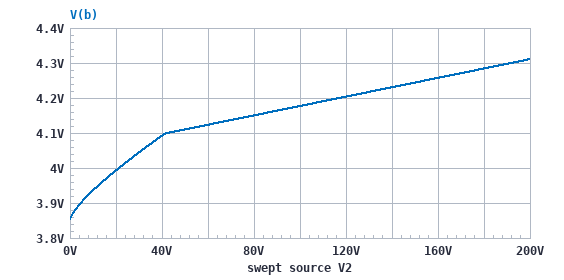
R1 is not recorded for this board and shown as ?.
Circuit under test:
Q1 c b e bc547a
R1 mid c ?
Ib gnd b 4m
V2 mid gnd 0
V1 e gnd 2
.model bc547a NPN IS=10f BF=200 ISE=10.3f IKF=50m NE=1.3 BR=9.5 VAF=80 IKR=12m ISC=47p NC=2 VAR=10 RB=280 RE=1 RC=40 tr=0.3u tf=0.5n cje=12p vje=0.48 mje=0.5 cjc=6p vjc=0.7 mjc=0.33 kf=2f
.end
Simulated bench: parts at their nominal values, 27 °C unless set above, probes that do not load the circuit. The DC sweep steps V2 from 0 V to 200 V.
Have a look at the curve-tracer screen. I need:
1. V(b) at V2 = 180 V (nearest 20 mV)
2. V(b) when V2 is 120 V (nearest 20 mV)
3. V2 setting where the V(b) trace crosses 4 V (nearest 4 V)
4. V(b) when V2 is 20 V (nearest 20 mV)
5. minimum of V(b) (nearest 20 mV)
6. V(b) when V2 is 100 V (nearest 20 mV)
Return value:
4.28 V
4.20 V
20 V
4.00 V
3.86 V
4.18 V
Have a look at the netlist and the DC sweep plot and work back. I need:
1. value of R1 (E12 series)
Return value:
220 Ω
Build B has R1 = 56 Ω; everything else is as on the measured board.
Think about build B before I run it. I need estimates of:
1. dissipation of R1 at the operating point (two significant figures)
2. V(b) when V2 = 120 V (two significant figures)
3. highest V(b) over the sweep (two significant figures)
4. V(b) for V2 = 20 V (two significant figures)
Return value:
20 mW
4.3 V
4.4 V
4.1 V
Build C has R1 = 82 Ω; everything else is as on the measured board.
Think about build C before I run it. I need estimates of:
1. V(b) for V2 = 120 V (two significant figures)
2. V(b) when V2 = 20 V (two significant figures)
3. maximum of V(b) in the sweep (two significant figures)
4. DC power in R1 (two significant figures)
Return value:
4.3 V
4.1 V
4.4 V
21 mW
